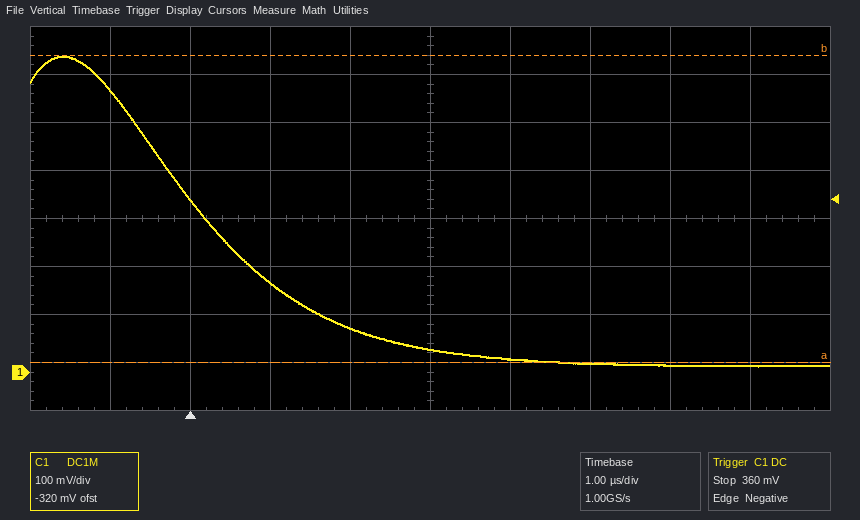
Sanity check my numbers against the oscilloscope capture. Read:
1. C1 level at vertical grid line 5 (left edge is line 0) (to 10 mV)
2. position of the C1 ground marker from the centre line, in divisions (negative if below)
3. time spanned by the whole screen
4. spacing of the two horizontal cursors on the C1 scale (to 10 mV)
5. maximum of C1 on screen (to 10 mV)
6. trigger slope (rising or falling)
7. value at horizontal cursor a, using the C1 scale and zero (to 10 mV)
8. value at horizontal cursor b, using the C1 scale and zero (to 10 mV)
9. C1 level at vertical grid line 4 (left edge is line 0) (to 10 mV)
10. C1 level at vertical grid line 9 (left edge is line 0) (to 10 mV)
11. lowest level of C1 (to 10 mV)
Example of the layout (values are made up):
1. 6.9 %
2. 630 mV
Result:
1. 50 mV
2. -3.2 div
3. 10 µs
4. 640 mV
5. 660 mV
6. falling
7. 20 mV
8. 660 mV
9. 90 mV
10. 10 mV
11. 10 mV
